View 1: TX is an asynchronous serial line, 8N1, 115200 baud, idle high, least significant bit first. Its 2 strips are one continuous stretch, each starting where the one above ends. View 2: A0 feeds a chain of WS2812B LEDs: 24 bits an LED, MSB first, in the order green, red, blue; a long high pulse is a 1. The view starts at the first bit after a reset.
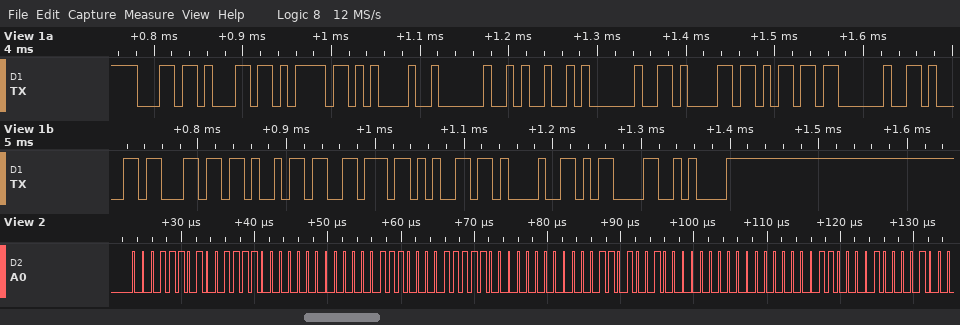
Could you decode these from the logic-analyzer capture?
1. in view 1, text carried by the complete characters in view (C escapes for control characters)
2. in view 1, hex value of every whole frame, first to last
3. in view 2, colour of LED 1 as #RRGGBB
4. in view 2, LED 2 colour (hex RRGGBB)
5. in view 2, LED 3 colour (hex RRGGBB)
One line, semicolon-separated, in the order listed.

"llo! I am alive!\r\n"; 6C 6C 6F 21 20 49 20 61 6D 20 61 6C 69 76 65 21 0D 0A; #3C1D00; #3E1C00; #401A00
